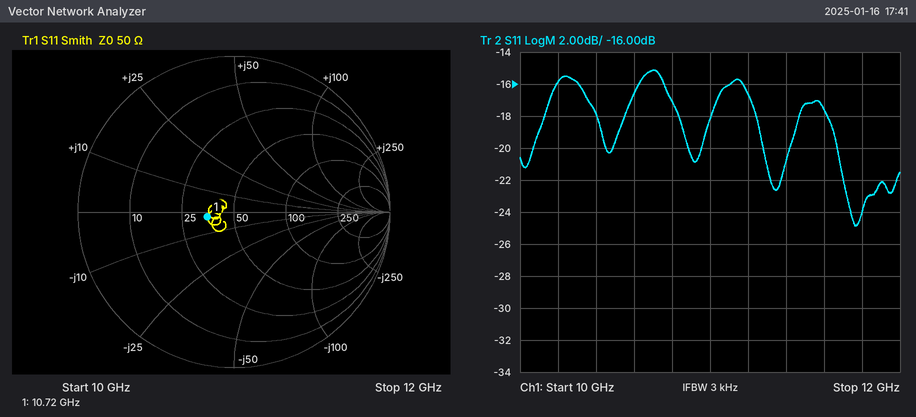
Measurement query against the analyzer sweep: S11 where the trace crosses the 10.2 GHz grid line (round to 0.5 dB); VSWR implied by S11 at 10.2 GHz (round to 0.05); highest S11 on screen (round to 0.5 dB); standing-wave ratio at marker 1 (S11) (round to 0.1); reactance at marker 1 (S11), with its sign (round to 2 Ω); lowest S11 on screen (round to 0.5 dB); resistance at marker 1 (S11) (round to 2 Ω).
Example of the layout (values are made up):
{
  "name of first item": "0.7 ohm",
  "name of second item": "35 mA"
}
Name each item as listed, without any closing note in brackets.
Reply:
{
  "S11 where the trace crosses the 10.2 GHz grid line": "-16.0 dB",
  "VSWR implied by S11 at 10.2 GHz": "1.40",
  "highest S11 on screen": "-15.0 dB",
  "standing-wave ratio at marker 1 (S11)": "1.4",
  "reactance at marker 1 (S11), with its sign": "-2 Ω",
  "lowest S11 on screen": "-25.0 dB",
  "resistance at marker 1 (S11)": "36 Ω"
}
